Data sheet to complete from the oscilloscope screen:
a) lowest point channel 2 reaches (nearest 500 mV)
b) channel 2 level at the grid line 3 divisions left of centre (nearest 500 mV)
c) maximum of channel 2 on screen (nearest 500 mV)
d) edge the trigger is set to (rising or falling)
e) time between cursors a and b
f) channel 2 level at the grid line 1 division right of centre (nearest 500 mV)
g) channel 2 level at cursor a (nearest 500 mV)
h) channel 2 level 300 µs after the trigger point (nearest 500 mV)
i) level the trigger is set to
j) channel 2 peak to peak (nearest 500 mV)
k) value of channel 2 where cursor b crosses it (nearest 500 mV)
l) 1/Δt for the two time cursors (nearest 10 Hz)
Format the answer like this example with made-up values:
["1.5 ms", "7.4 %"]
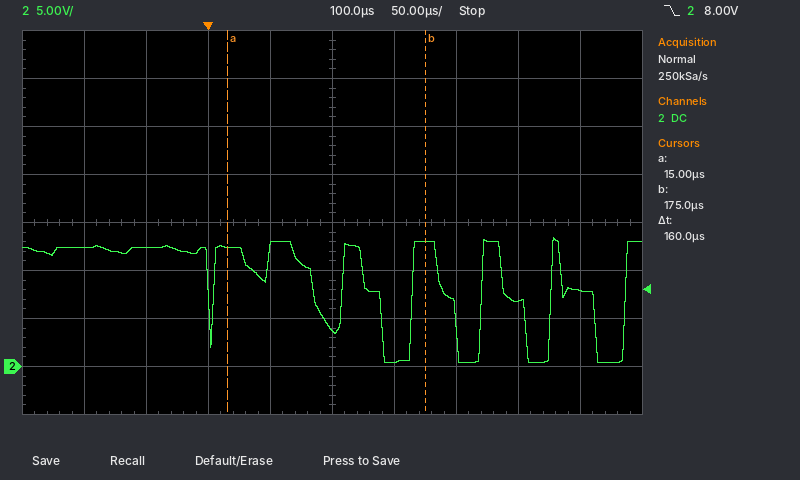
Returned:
["500 mV", "12.5 V", "13.5 V", "falling", "160 µs", "500 mV", "12.5 V", "8.0 V", "8.00 V", "13.0 V", "13.0 V", "6.25 kHz"]
